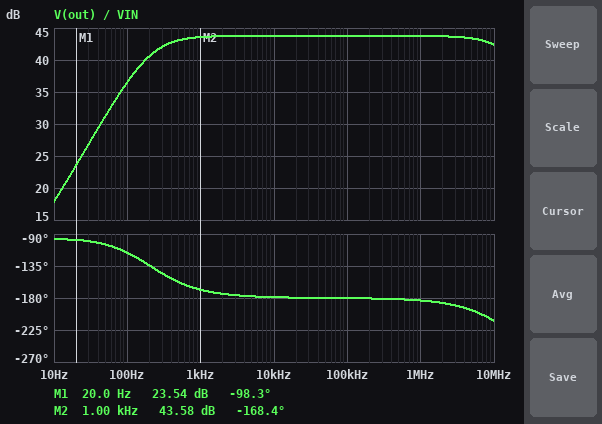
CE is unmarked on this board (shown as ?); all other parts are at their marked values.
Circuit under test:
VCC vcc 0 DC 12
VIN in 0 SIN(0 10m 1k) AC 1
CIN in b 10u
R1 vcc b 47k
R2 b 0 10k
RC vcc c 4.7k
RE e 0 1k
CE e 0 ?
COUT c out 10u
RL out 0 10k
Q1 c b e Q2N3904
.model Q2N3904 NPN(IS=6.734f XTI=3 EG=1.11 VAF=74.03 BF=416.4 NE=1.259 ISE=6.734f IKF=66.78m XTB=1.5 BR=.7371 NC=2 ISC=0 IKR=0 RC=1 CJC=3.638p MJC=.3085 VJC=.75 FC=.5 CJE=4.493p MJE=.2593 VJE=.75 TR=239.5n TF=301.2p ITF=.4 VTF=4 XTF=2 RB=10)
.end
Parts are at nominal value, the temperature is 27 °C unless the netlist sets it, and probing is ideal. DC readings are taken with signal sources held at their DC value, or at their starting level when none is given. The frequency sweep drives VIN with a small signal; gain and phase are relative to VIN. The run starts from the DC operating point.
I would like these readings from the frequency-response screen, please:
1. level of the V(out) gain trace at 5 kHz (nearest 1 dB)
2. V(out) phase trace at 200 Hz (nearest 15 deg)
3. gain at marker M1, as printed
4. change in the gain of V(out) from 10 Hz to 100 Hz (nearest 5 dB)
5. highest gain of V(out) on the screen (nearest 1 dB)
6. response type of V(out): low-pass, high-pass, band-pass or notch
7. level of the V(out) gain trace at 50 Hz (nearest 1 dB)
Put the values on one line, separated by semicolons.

44 dB; -135 deg; 23.54 dB; 20 dB; 44 dB; high-pass; 31 dB
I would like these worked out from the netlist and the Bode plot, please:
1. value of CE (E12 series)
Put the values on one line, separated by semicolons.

39 µF
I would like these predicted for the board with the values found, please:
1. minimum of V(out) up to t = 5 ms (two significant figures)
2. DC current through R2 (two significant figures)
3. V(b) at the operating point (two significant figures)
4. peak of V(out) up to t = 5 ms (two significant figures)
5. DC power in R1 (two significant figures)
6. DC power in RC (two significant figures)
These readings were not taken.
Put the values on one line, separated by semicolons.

-1.6 V; 200 µA; 2.0 V; 1.4 V; 2.1 mW; 8.5 mW
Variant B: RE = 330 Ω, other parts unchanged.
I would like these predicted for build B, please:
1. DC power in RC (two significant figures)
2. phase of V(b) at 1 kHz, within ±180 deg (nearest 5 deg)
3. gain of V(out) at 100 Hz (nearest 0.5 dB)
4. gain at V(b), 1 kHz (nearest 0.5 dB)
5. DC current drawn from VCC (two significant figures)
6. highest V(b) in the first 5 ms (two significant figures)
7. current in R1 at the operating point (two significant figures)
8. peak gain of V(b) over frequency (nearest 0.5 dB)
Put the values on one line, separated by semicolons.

26 mW; 25 deg; 6.0 dB; -1.5 dB; 2.6 mA; 1.5 V; 220 µA; 0 dB
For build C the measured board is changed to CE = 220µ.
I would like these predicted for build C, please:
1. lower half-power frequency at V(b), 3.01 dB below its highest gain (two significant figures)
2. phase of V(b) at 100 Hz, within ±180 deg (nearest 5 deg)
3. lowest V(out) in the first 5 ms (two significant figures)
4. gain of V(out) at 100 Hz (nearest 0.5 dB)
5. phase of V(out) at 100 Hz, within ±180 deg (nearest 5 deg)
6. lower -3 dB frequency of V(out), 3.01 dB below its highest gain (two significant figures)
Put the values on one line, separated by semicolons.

2.4 Hz; 5 deg; -1.7 V; 43.0 dB; -155 deg; 41 Hz
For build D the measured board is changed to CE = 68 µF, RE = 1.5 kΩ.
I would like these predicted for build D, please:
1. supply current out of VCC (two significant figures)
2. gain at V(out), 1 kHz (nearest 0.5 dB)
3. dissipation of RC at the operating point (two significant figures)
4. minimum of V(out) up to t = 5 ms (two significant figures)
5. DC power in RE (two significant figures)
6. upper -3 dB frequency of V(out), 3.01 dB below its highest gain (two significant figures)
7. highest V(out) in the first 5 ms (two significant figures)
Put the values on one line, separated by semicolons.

1.1 mA; 40.5 dB; 4.0 mW; -1.2 V; 1.3 mW; 20 MHz; 970 mV
